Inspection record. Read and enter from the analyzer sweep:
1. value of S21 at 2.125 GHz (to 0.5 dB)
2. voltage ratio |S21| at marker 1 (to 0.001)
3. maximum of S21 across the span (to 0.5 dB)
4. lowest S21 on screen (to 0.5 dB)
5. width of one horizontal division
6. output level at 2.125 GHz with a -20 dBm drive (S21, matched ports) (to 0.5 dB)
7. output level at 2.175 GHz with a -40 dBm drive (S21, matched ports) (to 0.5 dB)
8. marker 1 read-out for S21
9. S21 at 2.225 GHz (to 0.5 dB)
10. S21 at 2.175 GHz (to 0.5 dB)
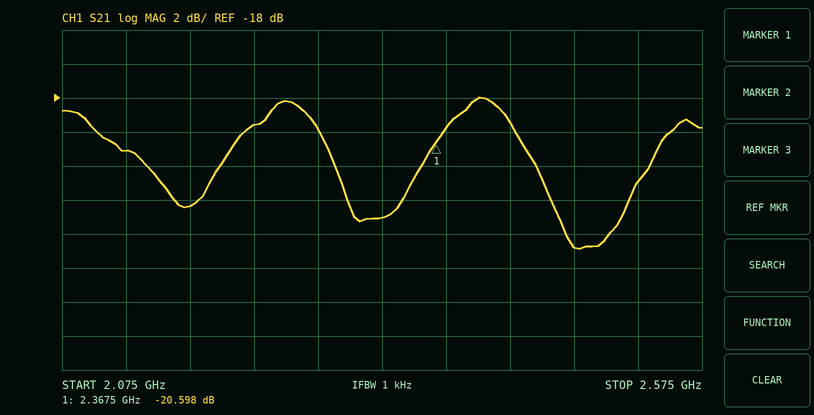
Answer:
-21.0 dB
0.093
-18.0 dB
-27.0 dB
50 MHz
-41.0 dBm
-64.5 dBm
-20.598 dB
-19.5 dB
-24.5 dB
